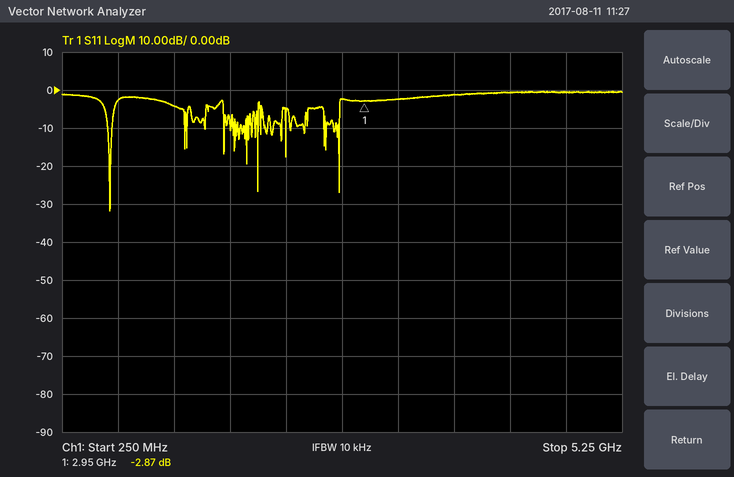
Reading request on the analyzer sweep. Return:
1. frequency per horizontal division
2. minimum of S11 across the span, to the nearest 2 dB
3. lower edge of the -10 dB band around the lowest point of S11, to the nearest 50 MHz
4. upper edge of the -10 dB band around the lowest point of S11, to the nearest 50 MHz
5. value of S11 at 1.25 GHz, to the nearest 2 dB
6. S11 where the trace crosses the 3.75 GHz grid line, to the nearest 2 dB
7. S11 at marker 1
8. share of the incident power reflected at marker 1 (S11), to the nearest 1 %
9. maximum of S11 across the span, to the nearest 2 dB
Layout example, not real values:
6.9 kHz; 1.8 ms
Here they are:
500 MHz; -32 dB; 650 MHz; 700 MHz; -4 dB; -2 dB; -2.87 dB; 52 %; 0 dB
